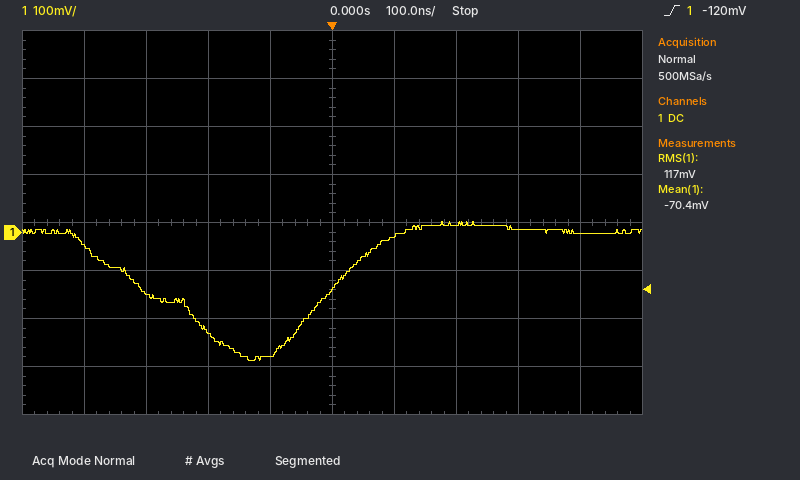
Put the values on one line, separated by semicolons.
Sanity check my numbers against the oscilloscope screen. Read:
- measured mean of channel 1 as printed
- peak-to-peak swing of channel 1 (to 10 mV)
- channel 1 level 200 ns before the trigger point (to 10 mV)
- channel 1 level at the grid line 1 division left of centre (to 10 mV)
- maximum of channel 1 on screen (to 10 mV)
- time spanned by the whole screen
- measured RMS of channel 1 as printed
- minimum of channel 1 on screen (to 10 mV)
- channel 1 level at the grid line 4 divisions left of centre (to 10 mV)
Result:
-70.4 mV; 290 mV; -210 mV; -260 mV; 20 mV; 1 µs; 117 mV; -270 mV; -30 mV
